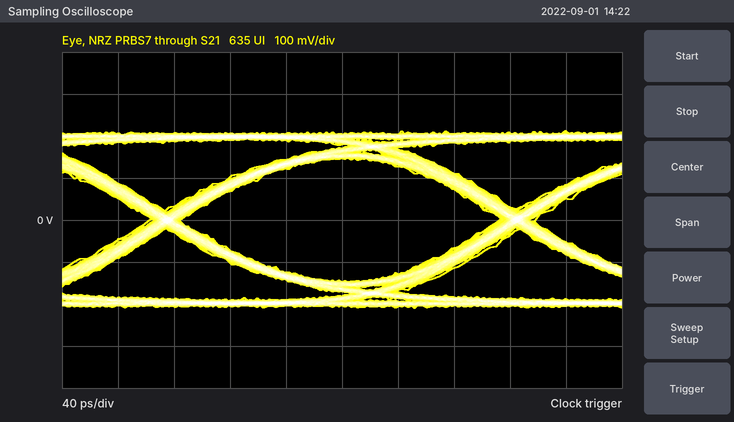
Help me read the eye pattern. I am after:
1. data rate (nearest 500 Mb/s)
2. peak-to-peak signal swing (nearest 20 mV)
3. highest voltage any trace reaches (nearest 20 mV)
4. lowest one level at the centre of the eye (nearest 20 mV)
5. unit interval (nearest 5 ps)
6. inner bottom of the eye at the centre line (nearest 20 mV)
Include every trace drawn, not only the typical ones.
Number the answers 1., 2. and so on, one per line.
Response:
1. 4.0 Gb/s
2. 420 mV
3. 220 mV
4. 140 mV
5. 250 ps
6. -140 mV
